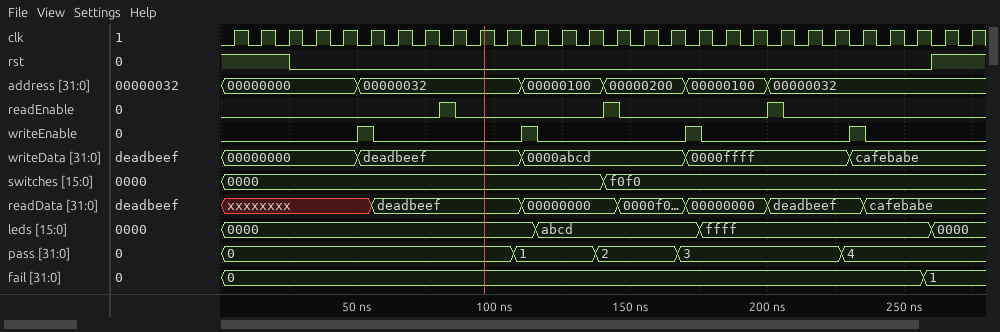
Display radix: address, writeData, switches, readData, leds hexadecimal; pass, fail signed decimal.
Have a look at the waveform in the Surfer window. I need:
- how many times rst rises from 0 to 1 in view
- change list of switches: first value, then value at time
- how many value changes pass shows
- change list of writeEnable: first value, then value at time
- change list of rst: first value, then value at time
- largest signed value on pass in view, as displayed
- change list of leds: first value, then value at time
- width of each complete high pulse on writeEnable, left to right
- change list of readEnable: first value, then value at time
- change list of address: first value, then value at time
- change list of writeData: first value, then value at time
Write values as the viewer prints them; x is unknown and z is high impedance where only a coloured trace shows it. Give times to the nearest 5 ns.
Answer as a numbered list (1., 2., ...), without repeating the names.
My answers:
1. 1
2. 0000, f0f0 at 140 ns
3. 4
4. 0, 1 at 50 ns, 0 at 55 ns, 1 at 110 ns, 0 at 115 ns, 1 at 170 ns, 0 at 175 ns, 1 at 230 ns, 0 at 235 ns
5. 1, 0 at 25 ns, 1 at 260 ns
6. 4
7. 0000, abcd at 115 ns, ffff at 175 ns, 0000 at 260 ns
8. 5 ns, 5 ns, 5 ns, 5 ns
9. 0, 1 at 80 ns, 0 at 85 ns, 1 at 140 ns, 0 at 145 ns, 1 at 200 ns, 0 at 205 ns
10. 00000000, 00000032 at 50 ns, 00000100 at 110 ns, 00000200 at 140 ns, 00000100 at 170 ns, 00000032 at 200 ns
11. 00000000, deadbeef at 50 ns, 0000abcd at 110 ns, 0000ffff at 170 ns, cafebabe at 230 ns
